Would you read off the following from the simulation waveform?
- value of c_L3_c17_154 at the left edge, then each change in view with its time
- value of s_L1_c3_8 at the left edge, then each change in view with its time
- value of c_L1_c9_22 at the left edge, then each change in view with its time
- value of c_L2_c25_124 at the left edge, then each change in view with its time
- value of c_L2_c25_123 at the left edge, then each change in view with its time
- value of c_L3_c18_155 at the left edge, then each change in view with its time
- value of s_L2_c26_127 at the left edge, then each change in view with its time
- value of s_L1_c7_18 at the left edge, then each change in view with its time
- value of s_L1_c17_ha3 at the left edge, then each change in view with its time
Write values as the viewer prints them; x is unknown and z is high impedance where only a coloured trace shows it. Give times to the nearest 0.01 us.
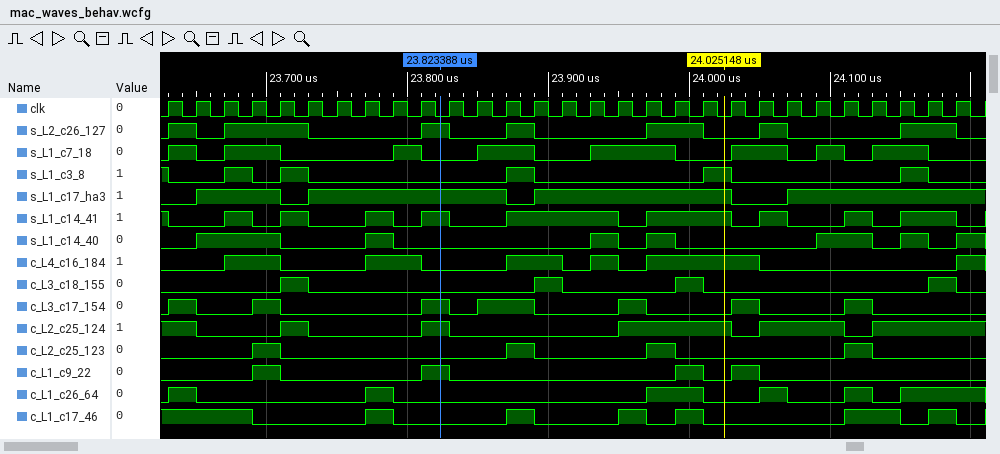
0, 1 at 23.63 us, 0 at 23.65 us, 1 at 23.69 us, 0 at 23.71 us, 1 at 23.81 us, 0 at 23.83 us, 1 at 23.85 us, 0 at 23.89 us, 1 at 23.95 us, 0 at 23.97 us, 1 at 24.03 us, 0 at 24.05 us, 1 at 24.11 us, 0 at 24.13 us
1, 0 at 23.63 us, 1 at 23.67 us, 0 at 23.69 us, 1 at 23.71 us, 0 at 23.73 us, 1 at 23.87 us, 0 at 23.89 us, 1 at 24.01 us, 0 at 24.03 us, 1 at 24.15 us, 0 at 24.17 us
0, 1 at 23.69 us, 0 at 23.71 us, 1 at 23.81 us, 0 at 23.83 us, 1 at 23.99 us, 0 at 24.01 us, 1 at 24.03 us, 0 at 24.05 us
1, 0 at 23.65 us, 1 at 23.71 us, 0 at 23.73 us, 1 at 23.81 us, 0 at 23.83 us, 1 at 23.95 us, 0 at 24.03 us, 1 at 24.05 us, 0 at 24.11 us, 1 at 24.13 us
0, 1 at 23.69 us, 0 at 23.71 us, 1 at 23.87 us, 0 at 23.89 us, 1 at 23.97 us, 0 at 23.99 us, 1 at 24.11 us, 0 at 24.13 us
0, 1 at 23.71 us, 0 at 23.73 us, 1 at 23.89 us, 0 at 23.91 us, 1 at 23.99 us, 0 at 24.01 us, 1 at 24.17 us, 0 at 24.19 us
0, 1 at 23.63 us, 0 at 23.65 us, 1 at 23.67 us, 0 at 23.73 us, 1 at 23.81 us, 0 at 23.83 us, 1 at 23.87 us, 0 at 23.89 us, 1 at 23.97 us, 0 at 24.01 us, 1 at 24.05 us, 0 at 24.07 us, 1 at 24.15 us, 0 at 24.19 us
0, 1 at 23.63 us, 0 at 23.65 us, 1 at 23.67 us, 0 at 23.71 us, 1 at 23.79 us, 0 at 23.81 us, 1 at 23.85 us, 0 at 23.89 us, 1 at 23.93 us, 0 at 23.99 us, 1 at 24.03 us, 0 at 24.07 us, 1 at 24.09 us, 0 at 24.11 us, 1 at 24.13 us, 0 at 24.17 us
0, 1 at 23.65 us, 0 at 23.71 us, 1 at 23.73 us, 0 at 23.87 us, 1 at 23.89 us, 0 at 24.03 us, 1 at 24.07 us
